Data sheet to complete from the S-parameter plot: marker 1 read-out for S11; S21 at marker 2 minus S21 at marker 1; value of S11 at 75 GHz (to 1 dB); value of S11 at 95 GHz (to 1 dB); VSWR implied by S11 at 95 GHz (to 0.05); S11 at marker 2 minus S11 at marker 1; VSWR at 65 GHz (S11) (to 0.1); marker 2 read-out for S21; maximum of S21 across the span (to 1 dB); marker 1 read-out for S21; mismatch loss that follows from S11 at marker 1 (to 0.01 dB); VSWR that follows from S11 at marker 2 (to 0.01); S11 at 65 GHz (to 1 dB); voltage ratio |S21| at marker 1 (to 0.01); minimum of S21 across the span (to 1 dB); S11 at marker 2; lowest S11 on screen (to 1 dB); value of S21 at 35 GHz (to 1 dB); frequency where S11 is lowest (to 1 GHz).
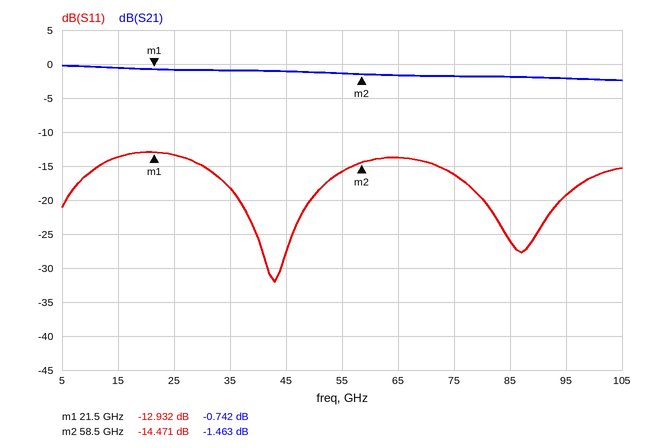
-12.932 dB
-0.721 dB
-16 dB
-19 dB
1.25
-1.539 dB
1.5
-1.463 dB
0 dB
-0.742 dB
0.23 dB
1.47
-14 dB
0.92
-2 dB
-14.471 dB
-32 dB
-1 dB
43 GHz
